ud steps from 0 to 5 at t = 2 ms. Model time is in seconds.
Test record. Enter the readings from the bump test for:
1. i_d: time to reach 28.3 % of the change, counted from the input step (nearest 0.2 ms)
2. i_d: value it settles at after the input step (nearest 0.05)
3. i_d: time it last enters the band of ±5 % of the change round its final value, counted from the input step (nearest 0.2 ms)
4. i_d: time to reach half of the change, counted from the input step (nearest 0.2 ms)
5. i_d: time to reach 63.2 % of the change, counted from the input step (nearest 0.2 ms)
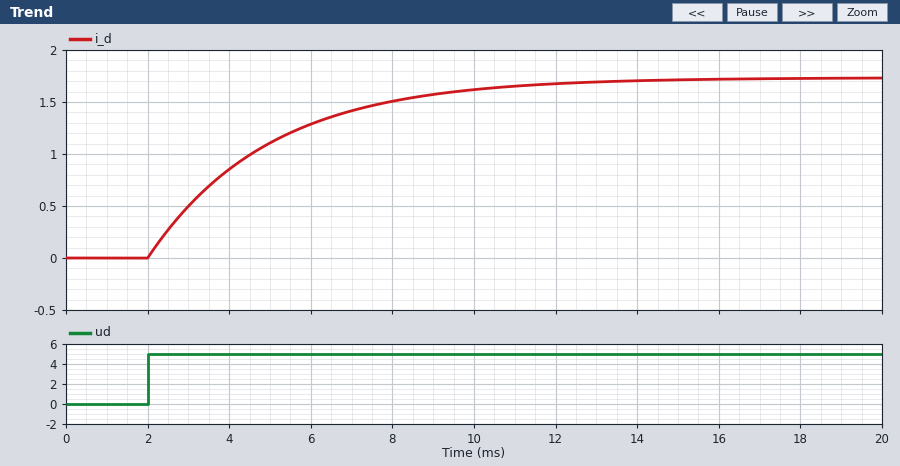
1.0 ms
1.75
8.8 ms
2.0 ms
3.0 ms
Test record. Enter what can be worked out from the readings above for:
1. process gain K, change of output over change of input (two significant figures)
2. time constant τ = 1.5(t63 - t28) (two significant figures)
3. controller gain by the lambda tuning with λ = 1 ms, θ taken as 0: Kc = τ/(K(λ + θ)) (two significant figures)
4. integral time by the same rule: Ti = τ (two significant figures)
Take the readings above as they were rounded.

0.35
3.0 ms
8.6
3.0 ms
